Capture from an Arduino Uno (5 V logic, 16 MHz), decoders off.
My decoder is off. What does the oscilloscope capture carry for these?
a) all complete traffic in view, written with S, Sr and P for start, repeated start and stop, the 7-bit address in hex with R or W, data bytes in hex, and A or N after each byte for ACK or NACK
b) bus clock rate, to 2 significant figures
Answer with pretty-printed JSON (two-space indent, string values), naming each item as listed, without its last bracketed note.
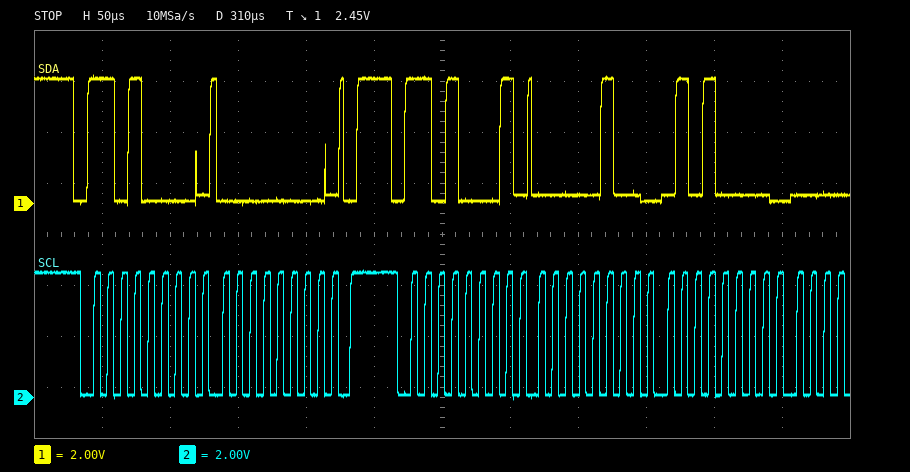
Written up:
{
  "all complete traffic in view, written with S, Sr and P for start, repeated start and stop, the 7-bit address in hex with R or W, data bytes in hex, and A or N after each byte for ACK or NACK": "S 68W A 00 A P S 68R A 04 A 50 A",
  "bus clock rate, to 2 significant figures": "100 kHz"
}
